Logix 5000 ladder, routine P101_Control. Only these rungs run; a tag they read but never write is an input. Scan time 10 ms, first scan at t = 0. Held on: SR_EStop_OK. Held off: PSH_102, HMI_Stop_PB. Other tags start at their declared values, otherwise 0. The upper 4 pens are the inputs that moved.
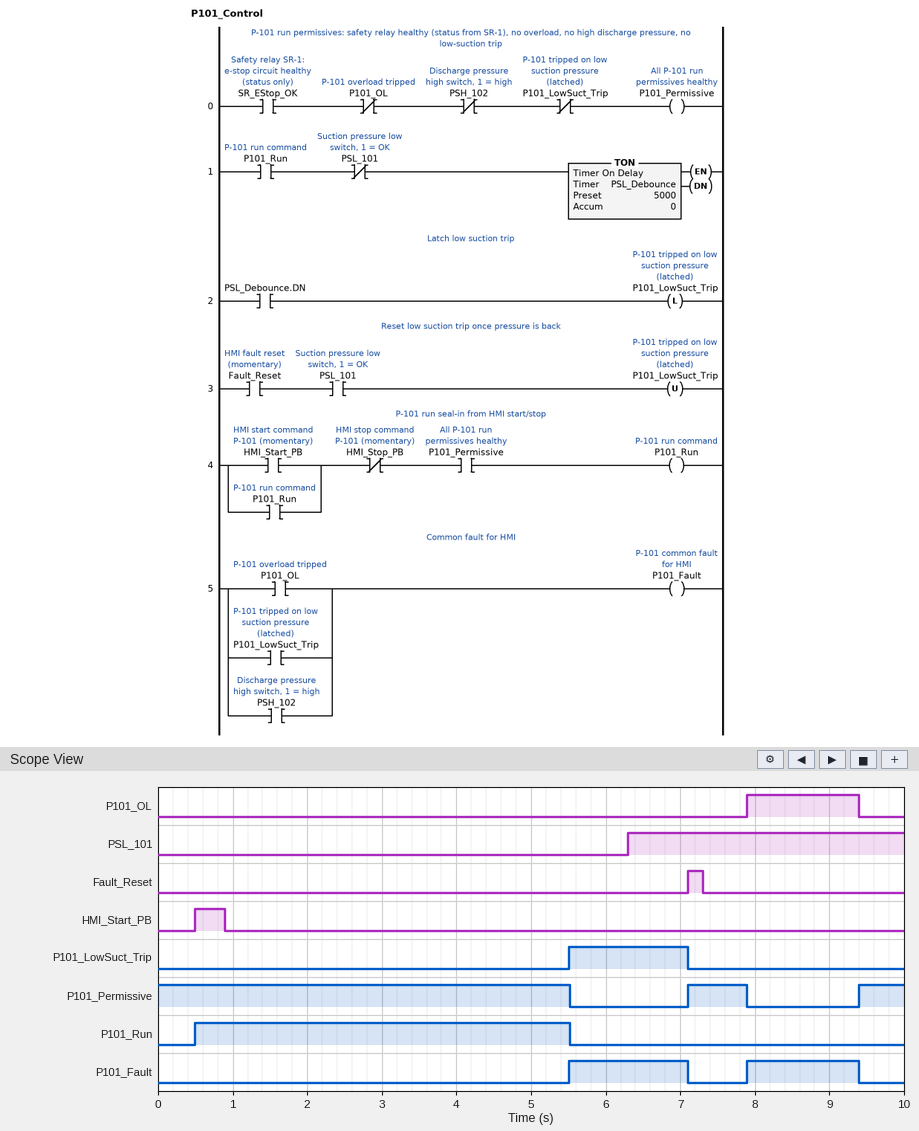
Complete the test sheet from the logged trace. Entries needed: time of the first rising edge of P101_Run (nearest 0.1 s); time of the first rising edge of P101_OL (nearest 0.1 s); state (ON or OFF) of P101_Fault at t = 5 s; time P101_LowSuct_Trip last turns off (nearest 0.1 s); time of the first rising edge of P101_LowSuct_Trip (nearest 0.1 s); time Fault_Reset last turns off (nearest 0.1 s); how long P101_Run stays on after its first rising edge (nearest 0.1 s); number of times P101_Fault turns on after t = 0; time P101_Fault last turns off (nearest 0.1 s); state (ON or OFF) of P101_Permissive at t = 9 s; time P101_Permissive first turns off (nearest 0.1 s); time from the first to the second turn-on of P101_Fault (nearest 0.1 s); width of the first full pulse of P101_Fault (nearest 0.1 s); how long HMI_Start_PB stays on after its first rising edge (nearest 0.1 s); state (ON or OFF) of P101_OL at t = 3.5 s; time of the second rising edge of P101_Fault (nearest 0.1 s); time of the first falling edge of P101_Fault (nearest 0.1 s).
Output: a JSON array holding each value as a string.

["0.5 s", "7.9 s", "OFF", "7.1 s", "5.5 s", "7.3 s", "5.0 s", "2", "9.4 s", "OFF", "5.5 s", "2.4 s", "1.6 s", "0.4 s", "OFF", "7.9 s", "7.1 s"]
